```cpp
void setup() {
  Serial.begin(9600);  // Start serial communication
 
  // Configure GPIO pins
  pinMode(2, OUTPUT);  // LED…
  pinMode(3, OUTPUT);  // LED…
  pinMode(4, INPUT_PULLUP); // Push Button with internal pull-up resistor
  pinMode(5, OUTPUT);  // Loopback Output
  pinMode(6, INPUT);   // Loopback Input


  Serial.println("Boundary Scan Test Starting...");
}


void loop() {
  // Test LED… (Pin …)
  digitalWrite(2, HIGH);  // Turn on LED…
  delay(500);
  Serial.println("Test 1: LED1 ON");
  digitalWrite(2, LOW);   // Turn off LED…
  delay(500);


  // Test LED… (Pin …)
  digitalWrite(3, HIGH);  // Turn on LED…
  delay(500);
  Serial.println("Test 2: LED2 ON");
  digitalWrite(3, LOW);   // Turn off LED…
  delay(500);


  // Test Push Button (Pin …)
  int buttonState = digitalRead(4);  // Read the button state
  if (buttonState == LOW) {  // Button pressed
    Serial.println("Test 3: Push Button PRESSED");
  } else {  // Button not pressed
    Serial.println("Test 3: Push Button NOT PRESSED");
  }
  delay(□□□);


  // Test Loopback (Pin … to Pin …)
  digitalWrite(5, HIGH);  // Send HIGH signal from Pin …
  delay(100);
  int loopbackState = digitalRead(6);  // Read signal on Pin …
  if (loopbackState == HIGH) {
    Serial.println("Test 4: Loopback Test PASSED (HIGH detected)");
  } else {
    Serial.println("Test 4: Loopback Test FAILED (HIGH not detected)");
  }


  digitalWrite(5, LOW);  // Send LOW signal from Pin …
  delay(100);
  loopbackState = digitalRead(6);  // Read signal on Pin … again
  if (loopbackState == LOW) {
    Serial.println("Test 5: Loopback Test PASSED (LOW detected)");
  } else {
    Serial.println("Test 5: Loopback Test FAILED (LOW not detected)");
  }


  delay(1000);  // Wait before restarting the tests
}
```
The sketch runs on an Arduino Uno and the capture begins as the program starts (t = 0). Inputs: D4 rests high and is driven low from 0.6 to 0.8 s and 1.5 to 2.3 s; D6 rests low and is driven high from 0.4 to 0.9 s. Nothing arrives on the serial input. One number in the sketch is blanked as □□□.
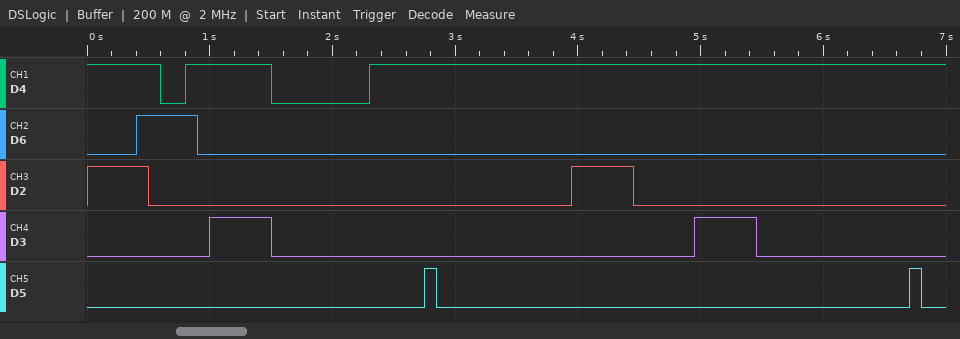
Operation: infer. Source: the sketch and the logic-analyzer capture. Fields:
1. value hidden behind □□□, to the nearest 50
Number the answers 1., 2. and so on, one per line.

1. 750
